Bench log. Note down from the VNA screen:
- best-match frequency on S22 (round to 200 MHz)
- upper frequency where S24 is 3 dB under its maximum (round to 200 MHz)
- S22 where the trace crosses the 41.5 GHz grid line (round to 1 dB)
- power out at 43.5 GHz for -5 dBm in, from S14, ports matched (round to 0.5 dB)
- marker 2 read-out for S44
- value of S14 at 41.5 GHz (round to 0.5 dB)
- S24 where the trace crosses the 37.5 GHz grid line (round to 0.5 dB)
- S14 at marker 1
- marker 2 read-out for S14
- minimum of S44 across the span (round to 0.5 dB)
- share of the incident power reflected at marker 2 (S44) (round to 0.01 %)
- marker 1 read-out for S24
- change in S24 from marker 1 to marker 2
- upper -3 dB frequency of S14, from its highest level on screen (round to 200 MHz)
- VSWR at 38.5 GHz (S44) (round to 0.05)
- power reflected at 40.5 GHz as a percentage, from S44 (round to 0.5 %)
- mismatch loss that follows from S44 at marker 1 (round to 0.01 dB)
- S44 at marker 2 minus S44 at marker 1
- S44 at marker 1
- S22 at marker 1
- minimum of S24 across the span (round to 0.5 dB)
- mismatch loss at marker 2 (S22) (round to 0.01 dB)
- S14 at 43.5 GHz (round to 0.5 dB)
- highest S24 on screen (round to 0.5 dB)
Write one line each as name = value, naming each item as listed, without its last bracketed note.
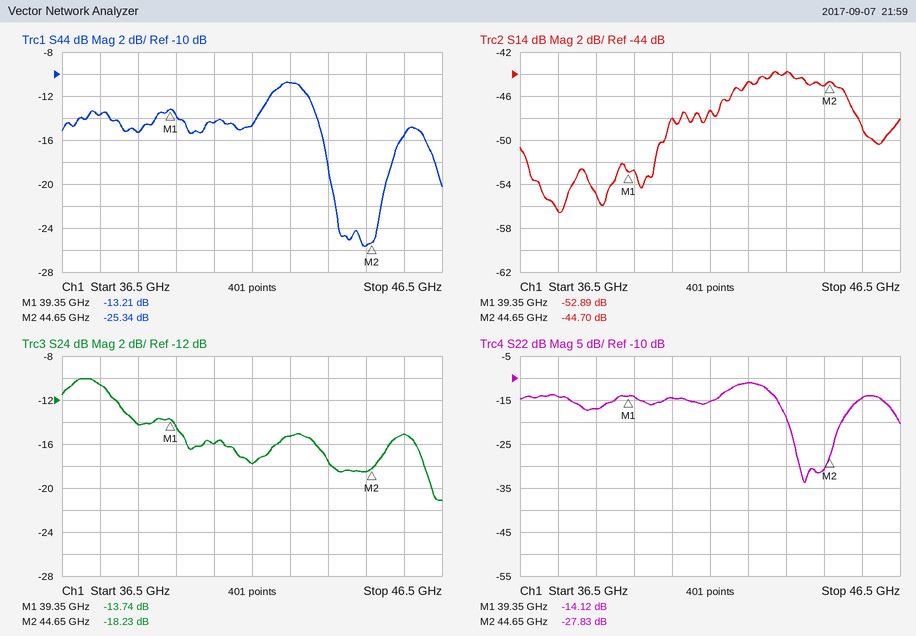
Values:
best-match frequency on S22 = 44.0 GHz
upper frequency where S24 is 3 dB under its maximum = 38.2 GHz
S22 where the trace crosses the 41.5 GHz grid line = -15 dB
power out at 43.5 GHz for -5 dBm in, from S14, ports matched = -49.0 dBm
marker 2 read-out for S44 = -25.34 dB
value of S14 at 41.5 GHz = -47.5 dB
S24 where the trace crosses the 37.5 GHz grid line = -10.5 dB
S14 at marker 1 = -52.89 dB
marker 2 read-out for S14 = -44.70 dB
minimum of S44 across the span = -25.5 dB
share of the incident power reflected at marker 2 (S44) = 0.29 %
marker 1 read-out for S24 = -13.74 dB
change in S24 from marker 1 to marker 2 = -4.49 dB
upper -3 dB frequency of S14, from its highest level on screen = 45.2 GHz
VSWR at 38.5 GHz (S44) = 1.40
power reflected at 40.5 GHz as a percentage, from S44 = 3.5 %
mismatch loss that follows from S44 at marker 1 = 0.21 dB
S44 at marker 2 minus S44 at marker 1 = -12.13 dB
S44 at marker 1 = -13.21 dB
S22 at marker 1 = -14.12 dB
minimum of S24 across the span = -21.0 dB
mismatch loss at marker 2 (S22) = 0.01 dB
S14 at 43.5 GHz = -44.0 dB
highest S24 on screen = -10.0 dB
